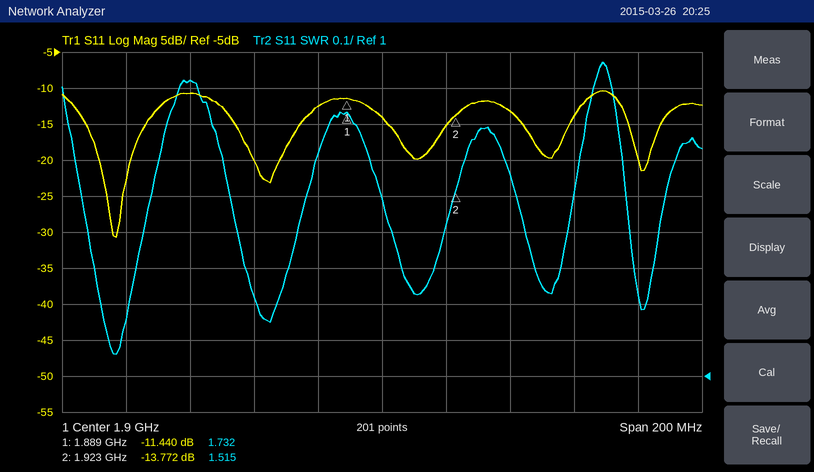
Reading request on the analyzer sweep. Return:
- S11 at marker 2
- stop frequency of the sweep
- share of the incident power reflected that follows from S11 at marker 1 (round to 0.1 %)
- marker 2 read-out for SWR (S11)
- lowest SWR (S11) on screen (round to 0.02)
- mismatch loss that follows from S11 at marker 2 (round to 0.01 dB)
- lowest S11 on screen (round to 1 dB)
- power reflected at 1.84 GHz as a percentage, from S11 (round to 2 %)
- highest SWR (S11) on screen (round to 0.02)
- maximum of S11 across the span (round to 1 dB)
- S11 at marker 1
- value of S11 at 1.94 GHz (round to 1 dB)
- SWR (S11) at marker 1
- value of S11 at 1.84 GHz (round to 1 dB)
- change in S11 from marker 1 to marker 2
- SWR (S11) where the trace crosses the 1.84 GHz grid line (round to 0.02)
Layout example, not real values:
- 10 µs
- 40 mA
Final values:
- -13.772 dB
- 2 GHz
- 7.2 %
- 1.515
- 1.06
- 0.19 dB
- -31 dB
- 8 %
- 1.88
- -10 dB
- -11.440 dB
- -13 dB
- 1.732
- -11 dB
- -2.332 dB
- 1.82
